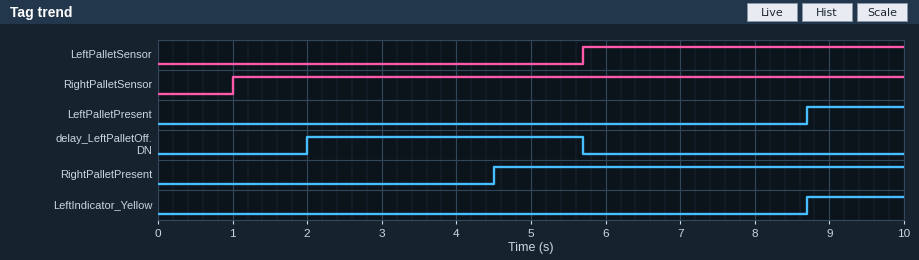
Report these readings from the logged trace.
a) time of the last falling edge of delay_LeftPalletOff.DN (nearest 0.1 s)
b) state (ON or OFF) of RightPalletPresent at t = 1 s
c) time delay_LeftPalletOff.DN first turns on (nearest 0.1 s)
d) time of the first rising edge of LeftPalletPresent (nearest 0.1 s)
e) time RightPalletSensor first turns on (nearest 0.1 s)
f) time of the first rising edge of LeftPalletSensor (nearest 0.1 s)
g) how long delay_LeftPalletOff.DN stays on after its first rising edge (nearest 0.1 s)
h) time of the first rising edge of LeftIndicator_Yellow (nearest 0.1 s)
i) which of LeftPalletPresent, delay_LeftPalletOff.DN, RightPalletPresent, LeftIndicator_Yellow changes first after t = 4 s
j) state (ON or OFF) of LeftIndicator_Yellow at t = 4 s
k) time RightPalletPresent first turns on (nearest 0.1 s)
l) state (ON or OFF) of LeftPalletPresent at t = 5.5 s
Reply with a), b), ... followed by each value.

a) 5.7 s
b) OFF
c) 2.0 s
d) 8.7 s
e) 1.0 s
f) 5.7 s
g) 3.7 s
h) 8.7 s
i) RightPalletPresent
j) OFF
k) 4.5 s
l) OFF
